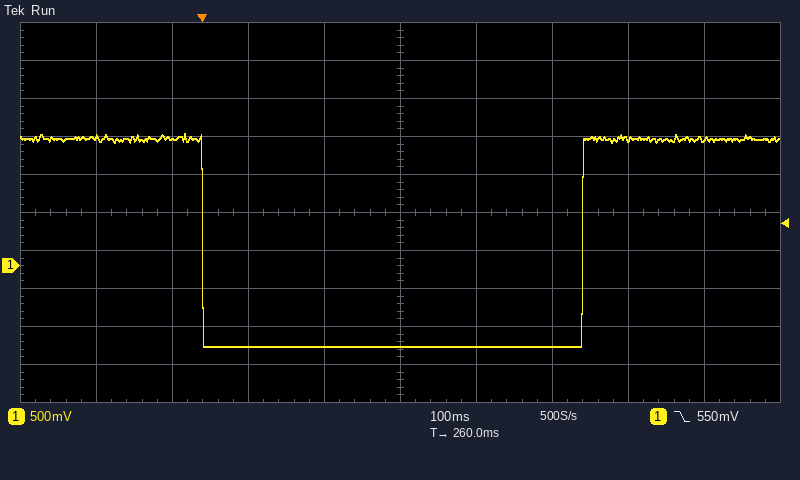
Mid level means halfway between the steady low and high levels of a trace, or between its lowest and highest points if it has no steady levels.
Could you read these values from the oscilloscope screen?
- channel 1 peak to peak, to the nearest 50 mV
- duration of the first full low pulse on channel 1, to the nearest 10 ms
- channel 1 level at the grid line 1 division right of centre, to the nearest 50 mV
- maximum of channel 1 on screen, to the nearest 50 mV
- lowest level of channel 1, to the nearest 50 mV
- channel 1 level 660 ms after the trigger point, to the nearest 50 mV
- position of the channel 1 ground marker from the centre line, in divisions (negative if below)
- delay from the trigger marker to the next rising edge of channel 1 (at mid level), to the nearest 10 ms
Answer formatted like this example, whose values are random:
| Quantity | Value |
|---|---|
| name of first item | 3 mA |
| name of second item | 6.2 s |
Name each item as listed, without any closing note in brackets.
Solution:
| Quantity | Value |
|---|---|
| channel 1 peak to peak, to the nearest 50 mV | 2.80 V |
| duration of the first full low pulse on channel 1, to the nearest 10 ms | 500 ms |
| channel 1 level at the grid line 1 division right of centre, to the nearest 50 mV | -1.05 V |
| maximum of channel 1 on screen, to the nearest 50 mV | 1.75 V |
| lowest level of channel 1, to the nearest 50 mV | -1.05 V |
| channel 1 level 660 ms after the trigger point, to the nearest 50 mV | 1.65 V |
| position of the channel 1 ground marker from the centre line, in divisions | -1.4 div |
| delay from the trigger marker to the next rising edge of channel 1 (at mid level), to the nearest 10 ms | 500 ms |
